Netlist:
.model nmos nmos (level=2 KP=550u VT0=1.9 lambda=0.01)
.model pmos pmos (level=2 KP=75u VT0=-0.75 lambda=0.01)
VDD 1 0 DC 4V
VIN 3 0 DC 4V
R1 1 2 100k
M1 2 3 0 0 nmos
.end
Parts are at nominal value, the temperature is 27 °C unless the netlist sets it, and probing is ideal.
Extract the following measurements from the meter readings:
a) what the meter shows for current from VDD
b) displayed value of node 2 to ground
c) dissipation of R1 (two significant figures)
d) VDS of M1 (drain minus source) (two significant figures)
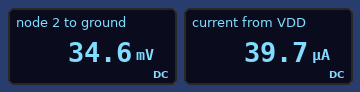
39.7 µA
34.6 mV
160 µW
35 mV
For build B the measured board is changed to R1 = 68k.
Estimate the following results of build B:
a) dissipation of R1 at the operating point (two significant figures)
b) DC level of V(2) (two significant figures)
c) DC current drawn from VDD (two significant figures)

230 µW
51 mV
58 µA
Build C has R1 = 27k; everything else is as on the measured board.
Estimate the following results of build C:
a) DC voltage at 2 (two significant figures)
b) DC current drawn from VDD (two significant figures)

130 mV
140 µA
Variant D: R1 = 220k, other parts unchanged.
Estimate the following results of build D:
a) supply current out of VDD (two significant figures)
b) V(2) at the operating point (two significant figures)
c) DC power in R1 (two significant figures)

18 µA
16 mV
72 µW
